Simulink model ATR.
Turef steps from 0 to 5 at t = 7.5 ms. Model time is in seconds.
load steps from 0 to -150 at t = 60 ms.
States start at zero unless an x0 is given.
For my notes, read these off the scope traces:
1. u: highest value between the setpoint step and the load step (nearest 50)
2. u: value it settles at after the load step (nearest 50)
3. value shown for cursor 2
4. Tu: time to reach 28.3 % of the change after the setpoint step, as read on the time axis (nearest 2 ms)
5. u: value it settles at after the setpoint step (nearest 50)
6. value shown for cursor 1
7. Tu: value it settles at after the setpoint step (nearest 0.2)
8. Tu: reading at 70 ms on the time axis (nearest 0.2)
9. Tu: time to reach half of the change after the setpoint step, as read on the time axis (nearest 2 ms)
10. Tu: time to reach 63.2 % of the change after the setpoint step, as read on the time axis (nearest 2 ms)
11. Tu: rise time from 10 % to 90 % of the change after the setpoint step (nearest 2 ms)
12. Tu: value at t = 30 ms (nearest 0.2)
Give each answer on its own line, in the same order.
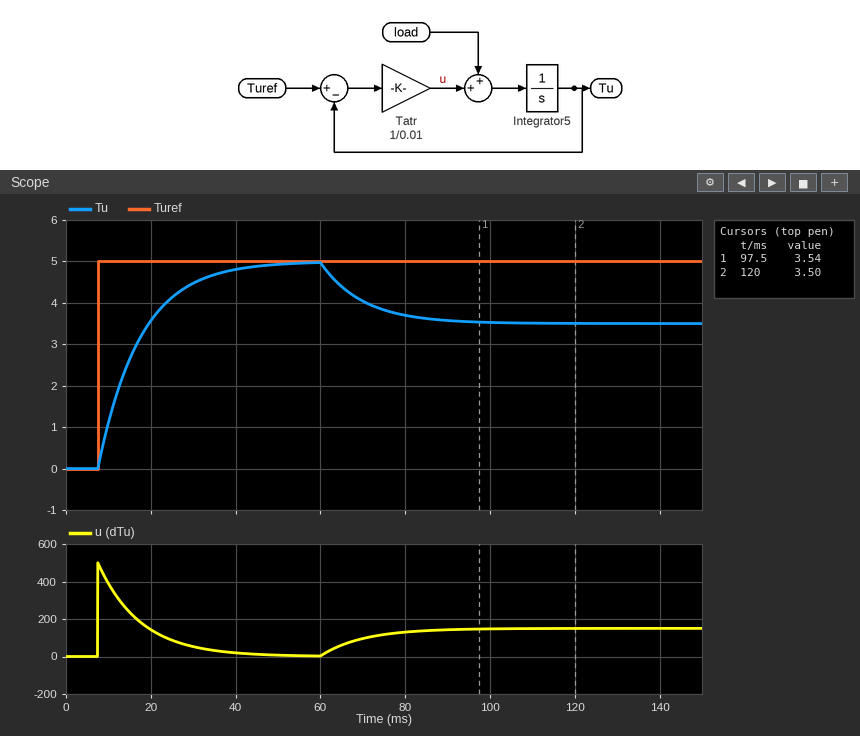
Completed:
500
150
3.50
10 ms
0
3.54
5.0
4.0
14 ms
18 ms
22 ms
4.4
